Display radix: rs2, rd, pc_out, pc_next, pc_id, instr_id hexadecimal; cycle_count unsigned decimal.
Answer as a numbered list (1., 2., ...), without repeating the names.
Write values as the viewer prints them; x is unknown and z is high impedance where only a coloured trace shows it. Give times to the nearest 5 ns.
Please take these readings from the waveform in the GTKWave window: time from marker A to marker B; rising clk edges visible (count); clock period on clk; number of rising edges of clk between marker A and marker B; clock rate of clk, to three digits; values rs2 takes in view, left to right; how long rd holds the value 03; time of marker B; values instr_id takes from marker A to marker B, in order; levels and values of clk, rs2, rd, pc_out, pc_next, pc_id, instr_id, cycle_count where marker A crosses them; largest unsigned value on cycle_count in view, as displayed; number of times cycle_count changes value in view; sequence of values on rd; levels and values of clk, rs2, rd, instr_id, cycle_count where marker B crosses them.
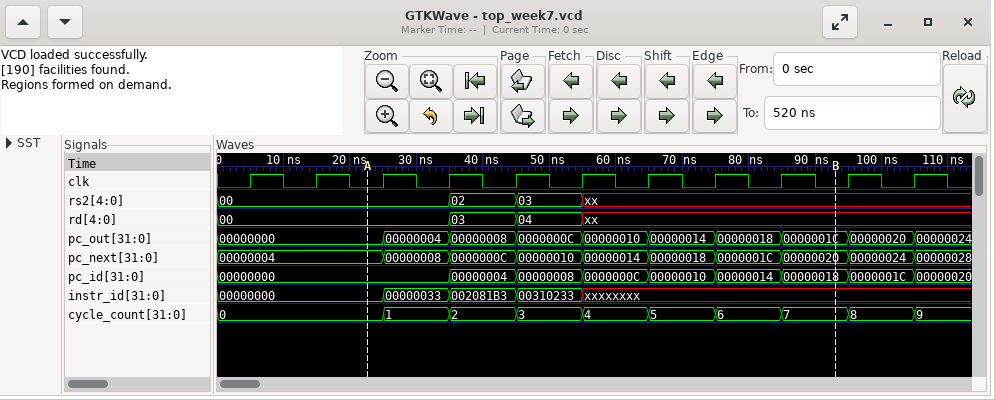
1. 70 ns
2. 11
3. 10 ns
4. 7
5. 100 MHz
6. 00, 02, 03, xx
7. 10 ns
8. 95 ns
9. 00000000, 00000033, 002081B3, 00310233, xxxxxxxx
10. clk=0, rs2=00, rd=00, pc_out=00000000, pc_next=00000004, pc_id=00000000, instr_id=00000000, cycle_count=0
11. 9
12. 9
13. 00, 03, 04, xx
14. clk=0, rs2=xx, rd=xx, instr_id=xxxxxxxx, cycle_count=7
